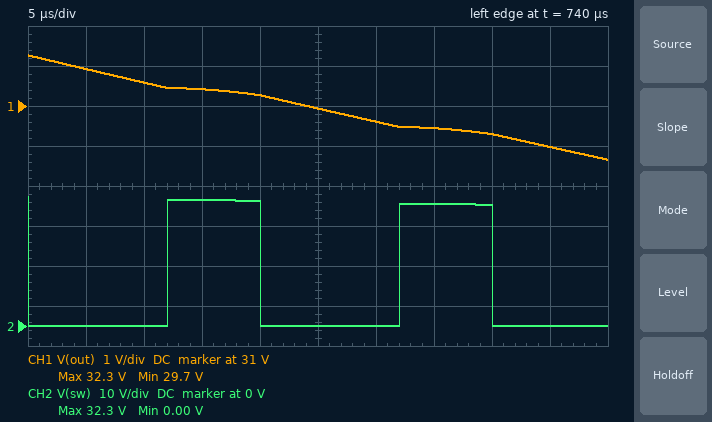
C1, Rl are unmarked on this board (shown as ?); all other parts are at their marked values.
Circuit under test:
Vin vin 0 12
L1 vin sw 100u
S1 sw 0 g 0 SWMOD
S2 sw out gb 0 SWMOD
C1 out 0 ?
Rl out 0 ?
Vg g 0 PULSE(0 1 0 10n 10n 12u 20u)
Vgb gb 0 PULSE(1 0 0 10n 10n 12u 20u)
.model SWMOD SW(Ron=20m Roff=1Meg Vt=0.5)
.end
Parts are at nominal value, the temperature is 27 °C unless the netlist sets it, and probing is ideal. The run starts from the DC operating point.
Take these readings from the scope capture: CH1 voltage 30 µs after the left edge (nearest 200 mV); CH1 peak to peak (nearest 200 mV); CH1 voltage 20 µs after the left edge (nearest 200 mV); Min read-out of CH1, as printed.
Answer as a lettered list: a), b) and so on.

a) 30.6 V
b) 2.6 V
c) 31.2 V
d) 29.7 V
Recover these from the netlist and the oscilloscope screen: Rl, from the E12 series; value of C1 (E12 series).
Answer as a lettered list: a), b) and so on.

a) 12 Ω
b) 39 µF
